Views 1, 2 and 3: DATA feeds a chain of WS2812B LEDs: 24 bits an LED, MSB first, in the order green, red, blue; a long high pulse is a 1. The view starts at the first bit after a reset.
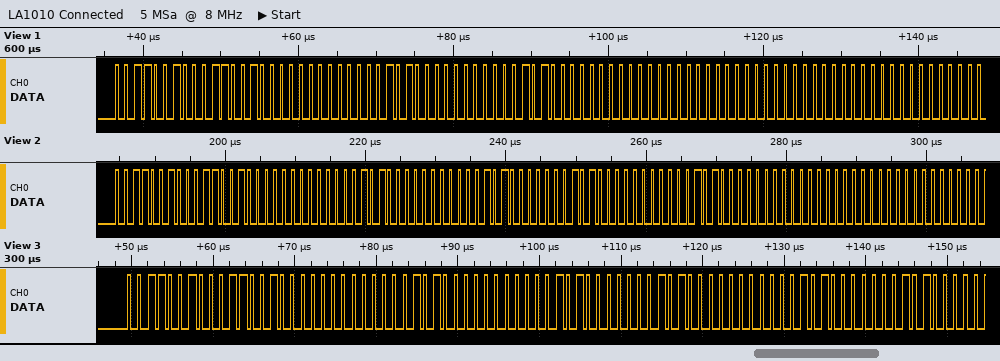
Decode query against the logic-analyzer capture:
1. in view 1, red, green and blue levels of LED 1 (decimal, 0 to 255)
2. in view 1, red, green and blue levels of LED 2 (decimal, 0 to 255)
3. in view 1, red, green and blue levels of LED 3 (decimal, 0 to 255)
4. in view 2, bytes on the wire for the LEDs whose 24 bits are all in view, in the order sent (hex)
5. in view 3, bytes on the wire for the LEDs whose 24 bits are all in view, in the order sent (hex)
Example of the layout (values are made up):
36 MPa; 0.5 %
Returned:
50, 50, 0; 0, 10, 40; 0, 0, 0; 32 32 00 0A 00 28 0A 00 28 00 00 00; 32 32 00 0A 00 28 0A 00 28
